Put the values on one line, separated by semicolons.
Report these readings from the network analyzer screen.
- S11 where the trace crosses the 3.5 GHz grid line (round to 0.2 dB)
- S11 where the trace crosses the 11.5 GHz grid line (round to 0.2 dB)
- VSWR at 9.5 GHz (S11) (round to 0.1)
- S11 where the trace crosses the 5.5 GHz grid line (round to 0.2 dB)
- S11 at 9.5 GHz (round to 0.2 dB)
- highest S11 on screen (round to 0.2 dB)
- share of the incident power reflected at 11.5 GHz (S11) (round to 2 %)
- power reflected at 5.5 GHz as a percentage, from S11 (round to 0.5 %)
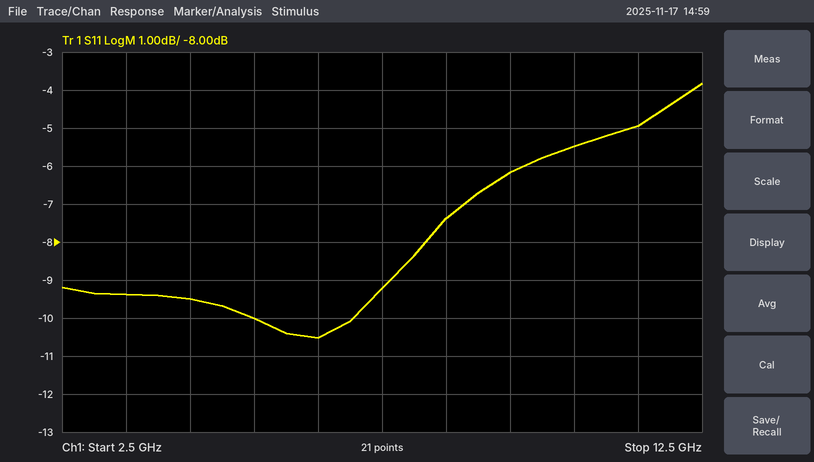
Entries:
-9.4 dB; -5.0 dB; 2.9; -10.0 dB; -6.2 dB; -3.8 dB; 32 %; 10.0 %
